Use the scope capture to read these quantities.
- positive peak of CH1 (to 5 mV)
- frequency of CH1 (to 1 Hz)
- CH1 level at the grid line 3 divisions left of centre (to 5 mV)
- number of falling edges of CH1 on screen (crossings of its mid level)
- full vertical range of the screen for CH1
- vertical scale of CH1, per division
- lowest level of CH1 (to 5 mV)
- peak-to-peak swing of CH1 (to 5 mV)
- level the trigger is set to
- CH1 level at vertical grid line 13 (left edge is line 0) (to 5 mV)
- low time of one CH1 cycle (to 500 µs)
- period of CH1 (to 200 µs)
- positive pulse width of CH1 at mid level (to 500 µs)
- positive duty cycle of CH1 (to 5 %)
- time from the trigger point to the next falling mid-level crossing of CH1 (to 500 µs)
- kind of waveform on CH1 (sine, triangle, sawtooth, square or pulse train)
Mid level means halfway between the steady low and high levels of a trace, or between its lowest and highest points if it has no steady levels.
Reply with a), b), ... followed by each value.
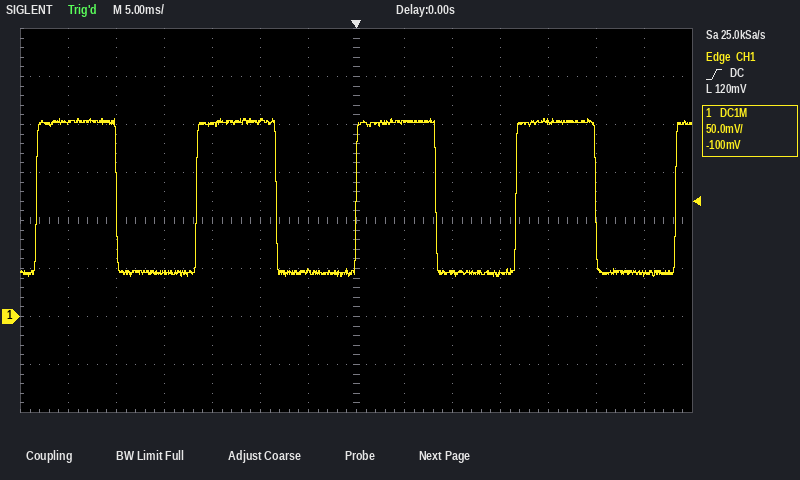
a) 205 mV
b) 60 Hz
c) 200 mV
d) 4
e) 400 mV
f) 50 mV
g) 40 mV
h) 165 mV
i) 120 mV
j) 45 mV
k) 8.5 ms
l) 16.6 ms
m) 8.5 ms
n) 50 %
o) 8.5 ms
p) square
